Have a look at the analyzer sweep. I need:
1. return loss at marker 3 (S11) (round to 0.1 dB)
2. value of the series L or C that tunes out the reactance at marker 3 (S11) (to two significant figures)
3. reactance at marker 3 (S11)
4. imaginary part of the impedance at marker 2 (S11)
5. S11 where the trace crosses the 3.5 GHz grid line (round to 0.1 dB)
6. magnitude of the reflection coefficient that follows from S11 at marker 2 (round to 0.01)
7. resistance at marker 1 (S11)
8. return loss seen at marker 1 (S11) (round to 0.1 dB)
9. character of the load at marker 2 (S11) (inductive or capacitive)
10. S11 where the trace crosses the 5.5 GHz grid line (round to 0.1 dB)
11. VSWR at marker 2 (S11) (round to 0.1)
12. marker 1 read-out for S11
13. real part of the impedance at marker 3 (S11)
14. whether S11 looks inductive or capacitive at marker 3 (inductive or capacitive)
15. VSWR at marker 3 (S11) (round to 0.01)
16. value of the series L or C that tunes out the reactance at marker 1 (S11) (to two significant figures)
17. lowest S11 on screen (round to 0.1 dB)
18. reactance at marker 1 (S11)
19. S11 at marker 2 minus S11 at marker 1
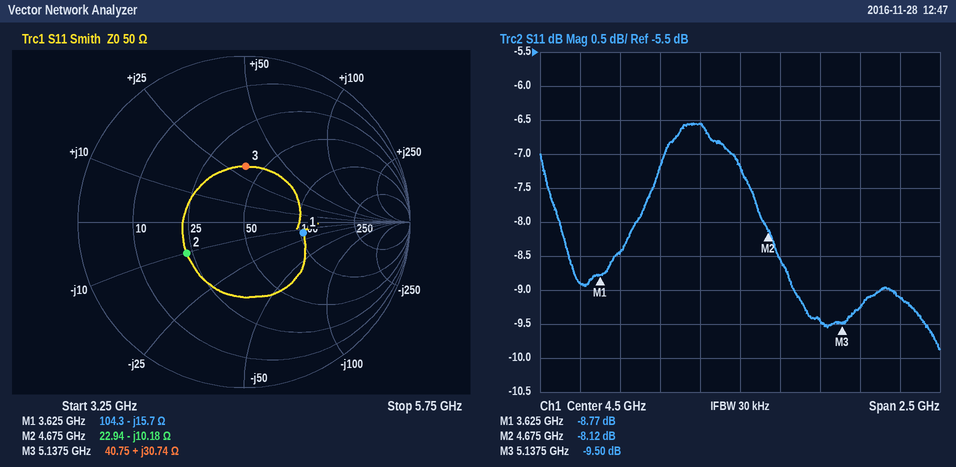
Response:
9.5 dB
1.0 pF
+30.74 Ω
-10.18 Ω
-8.9 dB
0.39
104.3 Ω
8.8 dB
capacitive
-9.1 dB
2.3
-8.77 dB
40.75 Ω
inductive
2.01
690 pH
-9.9 dB
-15.7 Ω
0.65 dB
